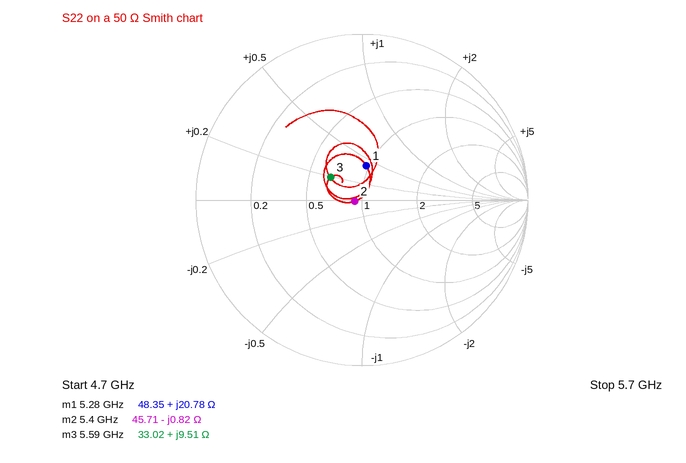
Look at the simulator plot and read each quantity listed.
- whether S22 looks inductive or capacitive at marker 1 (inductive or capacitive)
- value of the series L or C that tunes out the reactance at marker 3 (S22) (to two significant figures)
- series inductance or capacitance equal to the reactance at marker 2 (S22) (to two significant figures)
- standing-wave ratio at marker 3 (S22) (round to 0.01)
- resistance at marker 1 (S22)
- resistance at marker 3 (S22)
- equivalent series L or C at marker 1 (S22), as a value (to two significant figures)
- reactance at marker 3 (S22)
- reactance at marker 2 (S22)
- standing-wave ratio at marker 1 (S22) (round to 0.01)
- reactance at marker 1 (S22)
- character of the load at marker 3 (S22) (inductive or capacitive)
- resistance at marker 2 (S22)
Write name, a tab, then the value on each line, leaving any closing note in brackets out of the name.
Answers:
whether S22 looks inductive or capacitive at marker 1	inductive
value of the series L or C that tunes out the reactance at marker 3 (S22)	3.0 pF
series inductance or capacitance equal to the reactance at marker 2 (S22)	36 pF
standing-wave ratio at marker 3 (S22)	1.61
resistance at marker 1	48.35 Ω
resistance at marker 3	33.02 Ω
equivalent series L or C at marker 1 (S22), as a value	630 pH
reactance at marker 3	+9.51 Ω
reactance at marker 2	-0.82 Ω
standing-wave ratio at marker 1 (S22)	1.52
reactance at marker 1	+20.78 Ω
character of the load at marker 3 (S22)	inductive
resistance at marker 2	45.71 Ω
